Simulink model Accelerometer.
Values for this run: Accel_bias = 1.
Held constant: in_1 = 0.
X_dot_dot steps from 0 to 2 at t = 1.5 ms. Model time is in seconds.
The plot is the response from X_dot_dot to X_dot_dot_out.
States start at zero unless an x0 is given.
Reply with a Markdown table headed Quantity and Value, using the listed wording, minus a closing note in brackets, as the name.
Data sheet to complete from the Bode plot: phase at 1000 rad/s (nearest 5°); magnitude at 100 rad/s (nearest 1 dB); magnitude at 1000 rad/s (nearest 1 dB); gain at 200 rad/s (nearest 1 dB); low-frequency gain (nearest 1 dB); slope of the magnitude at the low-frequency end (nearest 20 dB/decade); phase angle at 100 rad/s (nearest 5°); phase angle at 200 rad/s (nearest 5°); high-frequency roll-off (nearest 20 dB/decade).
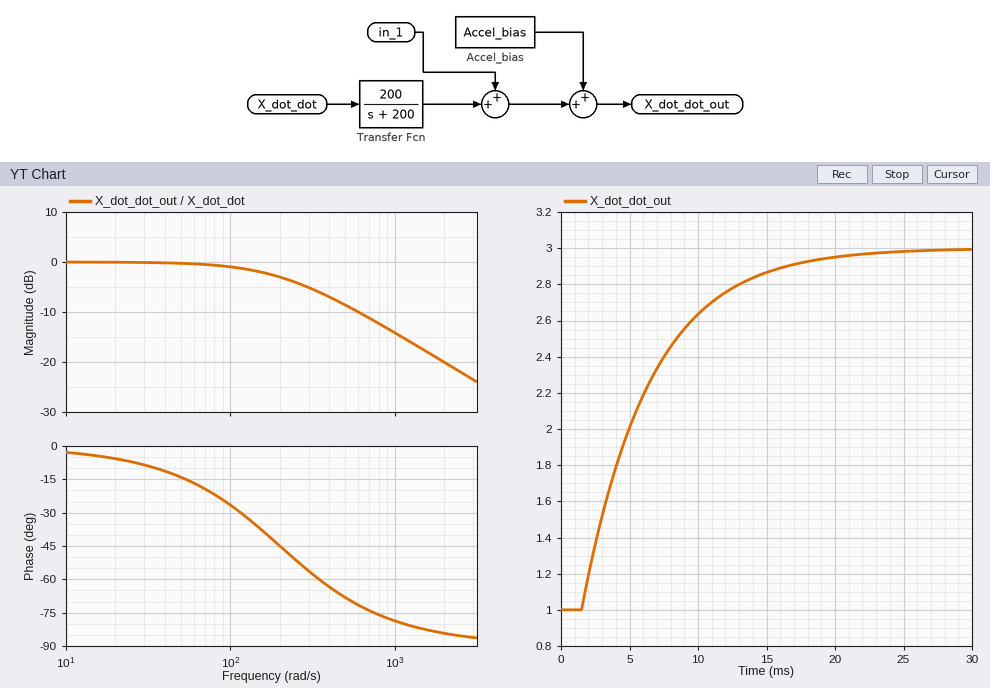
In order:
| Quantity | Value |
|---|---|
| phase at 1000 rad/s | -80° |
| magnitude at 100 rad/s | -1 dB |
| magnitude at 1000 rad/s | -14 dB |
| gain at 200 rad/s | -3 dB |
| low-frequency gain | 0 dB |
| slope of the magnitude at the low-frequency end | 0 dB/decade |
| phase angle at 100 rad/s | -25° |
| phase angle at 200 rad/s | -45° |
| high-frequency roll-off | -20 dB/decade |
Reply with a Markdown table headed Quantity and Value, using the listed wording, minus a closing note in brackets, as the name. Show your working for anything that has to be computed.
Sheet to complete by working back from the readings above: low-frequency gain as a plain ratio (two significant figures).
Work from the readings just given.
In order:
| Quantity | Value |
|---|---|
| low-frequency gain as a plain ratio | 10^(0 / 20) = 1.0 |
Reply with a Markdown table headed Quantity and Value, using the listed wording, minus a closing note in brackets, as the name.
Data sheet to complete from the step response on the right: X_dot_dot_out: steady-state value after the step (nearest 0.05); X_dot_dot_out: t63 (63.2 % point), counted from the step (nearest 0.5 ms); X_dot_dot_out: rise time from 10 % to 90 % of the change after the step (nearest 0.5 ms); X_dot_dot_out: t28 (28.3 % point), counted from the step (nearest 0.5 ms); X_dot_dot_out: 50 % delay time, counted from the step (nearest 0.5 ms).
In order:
| Quantity | Value |
|---|---|
| X_dot_dot_out: steady-state value after the step | 3.00 |
| X_dot_dot_out: t63 (63.2 % point), counted from the step | 5.0 ms |
| X_dot_dot_out: rise time from 10 % to 90 % of the change after the step | 11.0 ms |
| X_dot_dot_out: t28 (28.3 % point), counted from the step | 1.5 ms |
| X_dot_dot_out: 50 % delay time, counted from the step | 3.5 ms |
